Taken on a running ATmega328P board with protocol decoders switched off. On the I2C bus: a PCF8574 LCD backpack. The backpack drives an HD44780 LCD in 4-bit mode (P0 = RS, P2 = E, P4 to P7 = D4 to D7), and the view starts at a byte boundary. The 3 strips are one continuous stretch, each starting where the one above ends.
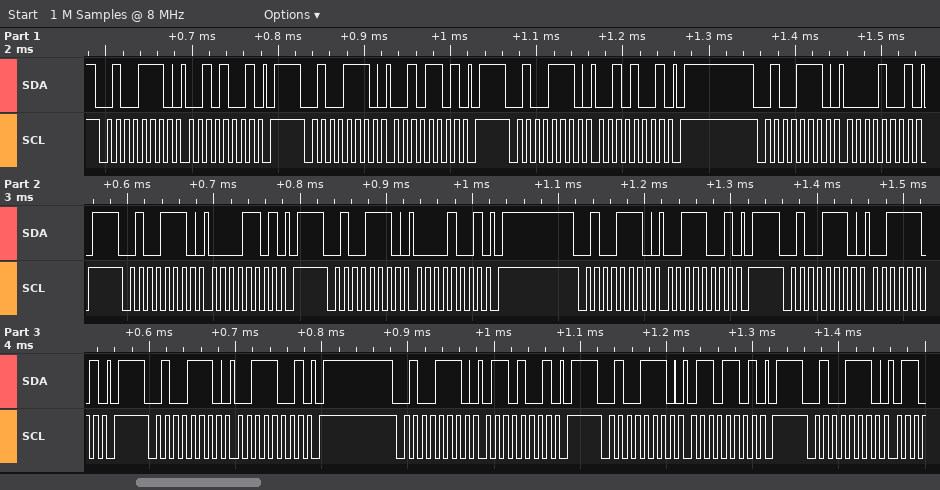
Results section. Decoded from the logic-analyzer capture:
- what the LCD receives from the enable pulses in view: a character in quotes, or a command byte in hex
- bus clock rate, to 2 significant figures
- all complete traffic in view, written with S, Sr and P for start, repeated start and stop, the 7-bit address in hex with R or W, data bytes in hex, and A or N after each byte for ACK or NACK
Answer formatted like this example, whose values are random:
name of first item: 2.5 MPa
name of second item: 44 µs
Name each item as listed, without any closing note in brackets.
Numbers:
what the LCD receives from the enable pulses in view: a character in quotes, or a command byte in hex: ' '
bus clock rate, to 2 significant figures: 100 kHz
all complete traffic in view, written with S, Sr and P for start, repeated start and stop, the 7-bit address in hex with R or W, data bytes in hex, and A or N after each byte for ACK or NACK: S 27W A 29 A P S 27W A 2D A P S 27W A 29 A P S 27W A 09 A P S 27W A 0D A P S 27W A 09 A P S 27W A 39 A P S 27W A 3D A P S 27W A 39 A P S 27W A 69 A P S 27W A 6D A P S 27W A
